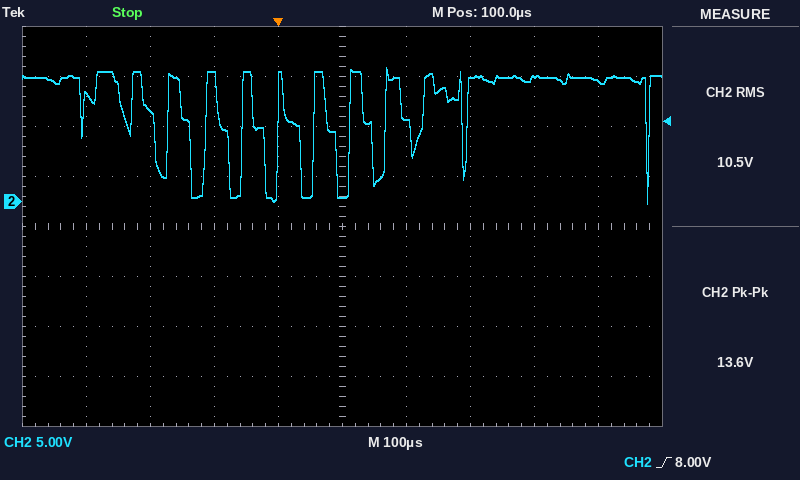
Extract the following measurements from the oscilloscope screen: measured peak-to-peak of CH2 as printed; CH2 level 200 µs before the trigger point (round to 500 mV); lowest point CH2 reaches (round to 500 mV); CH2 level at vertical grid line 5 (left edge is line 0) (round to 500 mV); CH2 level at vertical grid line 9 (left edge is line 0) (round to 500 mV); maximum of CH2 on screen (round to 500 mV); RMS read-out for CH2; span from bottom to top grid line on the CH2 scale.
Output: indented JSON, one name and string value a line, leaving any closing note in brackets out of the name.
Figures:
{
  "measured peak-to-peak of CH2 as printed": "13.6 V",
  "CH2 level 200 µs before the trigger point": "9.0 V",
  "lowest point CH2 reaches": "0.0 V",
  "CH2 level at vertical grid line 5 (left edge is line 0)": "500 mV",
  "CH2 level at vertical grid line 9 (left edge is line 0)": "12.0 V",
  "maximum of CH2 on screen": "13.5 V",
  "RMS read-out for CH2": "10.5 V",
  "span from bottom to top grid line on the CH2 scale": "40 V"
}
